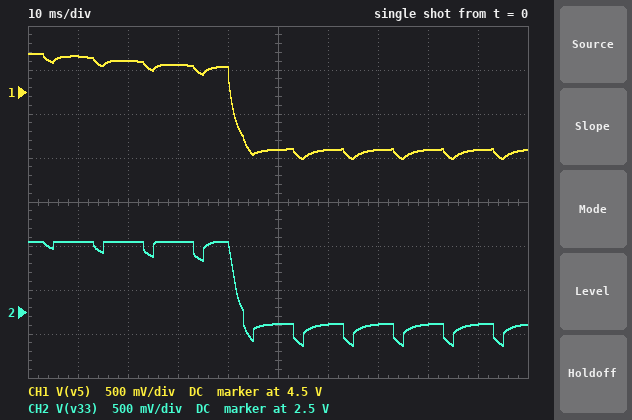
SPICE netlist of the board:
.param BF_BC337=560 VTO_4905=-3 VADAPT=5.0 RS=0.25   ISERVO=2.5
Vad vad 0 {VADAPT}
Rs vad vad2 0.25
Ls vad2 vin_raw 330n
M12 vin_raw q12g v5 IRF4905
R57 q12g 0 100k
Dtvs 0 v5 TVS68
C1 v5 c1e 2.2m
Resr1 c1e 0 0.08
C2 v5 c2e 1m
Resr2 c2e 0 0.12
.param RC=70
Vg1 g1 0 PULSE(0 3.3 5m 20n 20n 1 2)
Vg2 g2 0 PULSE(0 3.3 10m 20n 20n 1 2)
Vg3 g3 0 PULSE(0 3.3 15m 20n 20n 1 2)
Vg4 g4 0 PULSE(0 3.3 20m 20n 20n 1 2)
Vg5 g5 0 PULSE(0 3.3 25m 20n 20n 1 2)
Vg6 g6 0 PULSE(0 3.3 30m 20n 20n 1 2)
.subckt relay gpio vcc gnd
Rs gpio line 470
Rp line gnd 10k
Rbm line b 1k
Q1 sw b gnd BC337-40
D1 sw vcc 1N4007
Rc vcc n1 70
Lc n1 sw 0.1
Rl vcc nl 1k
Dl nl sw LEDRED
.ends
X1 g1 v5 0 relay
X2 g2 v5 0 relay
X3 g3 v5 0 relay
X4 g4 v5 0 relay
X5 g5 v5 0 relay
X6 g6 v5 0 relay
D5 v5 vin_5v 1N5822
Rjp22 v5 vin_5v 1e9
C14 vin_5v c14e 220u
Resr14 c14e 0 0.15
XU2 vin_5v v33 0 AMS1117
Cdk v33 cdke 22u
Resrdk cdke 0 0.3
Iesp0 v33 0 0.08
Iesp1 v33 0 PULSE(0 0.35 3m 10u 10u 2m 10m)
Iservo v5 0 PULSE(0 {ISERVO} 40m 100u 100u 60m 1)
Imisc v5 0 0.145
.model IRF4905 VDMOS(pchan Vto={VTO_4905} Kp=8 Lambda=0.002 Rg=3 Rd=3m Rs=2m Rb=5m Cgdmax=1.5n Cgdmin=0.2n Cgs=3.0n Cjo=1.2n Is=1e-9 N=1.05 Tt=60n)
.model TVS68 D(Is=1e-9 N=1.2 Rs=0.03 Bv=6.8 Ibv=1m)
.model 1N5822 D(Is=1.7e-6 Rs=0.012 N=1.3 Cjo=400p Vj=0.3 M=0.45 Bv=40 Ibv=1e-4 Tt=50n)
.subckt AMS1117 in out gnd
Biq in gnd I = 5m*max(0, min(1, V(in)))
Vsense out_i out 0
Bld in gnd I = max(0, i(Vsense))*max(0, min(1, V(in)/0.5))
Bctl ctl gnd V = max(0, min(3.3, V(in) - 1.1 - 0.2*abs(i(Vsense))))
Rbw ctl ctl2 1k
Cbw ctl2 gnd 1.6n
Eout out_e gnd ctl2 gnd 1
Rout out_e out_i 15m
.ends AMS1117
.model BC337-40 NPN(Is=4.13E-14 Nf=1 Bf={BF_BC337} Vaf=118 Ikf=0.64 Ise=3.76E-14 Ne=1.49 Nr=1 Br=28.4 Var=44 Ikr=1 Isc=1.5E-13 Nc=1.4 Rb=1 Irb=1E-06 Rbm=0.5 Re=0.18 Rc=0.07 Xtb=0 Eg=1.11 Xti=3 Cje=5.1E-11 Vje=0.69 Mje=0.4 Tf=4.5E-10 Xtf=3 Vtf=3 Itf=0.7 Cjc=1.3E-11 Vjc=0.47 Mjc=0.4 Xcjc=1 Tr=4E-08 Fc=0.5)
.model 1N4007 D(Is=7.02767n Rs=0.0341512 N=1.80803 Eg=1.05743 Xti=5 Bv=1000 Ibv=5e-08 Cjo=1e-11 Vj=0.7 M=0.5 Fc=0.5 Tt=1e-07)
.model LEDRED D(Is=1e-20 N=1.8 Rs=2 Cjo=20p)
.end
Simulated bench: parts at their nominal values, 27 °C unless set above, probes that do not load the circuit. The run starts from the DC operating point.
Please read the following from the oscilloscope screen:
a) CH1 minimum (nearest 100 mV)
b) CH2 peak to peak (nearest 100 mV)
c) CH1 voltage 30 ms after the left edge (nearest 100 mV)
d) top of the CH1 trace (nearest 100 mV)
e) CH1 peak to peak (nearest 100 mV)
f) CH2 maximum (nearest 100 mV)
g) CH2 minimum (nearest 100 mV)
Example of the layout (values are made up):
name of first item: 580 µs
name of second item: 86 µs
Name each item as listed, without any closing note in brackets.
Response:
CH1 minimum: 3.7 V
CH2 peak to peak: 1.2 V
CH1 voltage 30 ms after the left edge: 4.8 V
top of the CH1 trace: 4.9 V
CH1 peak to peak: 1.2 V
CH2 maximum: 3.3 V
CH2 minimum: 2.1 V
